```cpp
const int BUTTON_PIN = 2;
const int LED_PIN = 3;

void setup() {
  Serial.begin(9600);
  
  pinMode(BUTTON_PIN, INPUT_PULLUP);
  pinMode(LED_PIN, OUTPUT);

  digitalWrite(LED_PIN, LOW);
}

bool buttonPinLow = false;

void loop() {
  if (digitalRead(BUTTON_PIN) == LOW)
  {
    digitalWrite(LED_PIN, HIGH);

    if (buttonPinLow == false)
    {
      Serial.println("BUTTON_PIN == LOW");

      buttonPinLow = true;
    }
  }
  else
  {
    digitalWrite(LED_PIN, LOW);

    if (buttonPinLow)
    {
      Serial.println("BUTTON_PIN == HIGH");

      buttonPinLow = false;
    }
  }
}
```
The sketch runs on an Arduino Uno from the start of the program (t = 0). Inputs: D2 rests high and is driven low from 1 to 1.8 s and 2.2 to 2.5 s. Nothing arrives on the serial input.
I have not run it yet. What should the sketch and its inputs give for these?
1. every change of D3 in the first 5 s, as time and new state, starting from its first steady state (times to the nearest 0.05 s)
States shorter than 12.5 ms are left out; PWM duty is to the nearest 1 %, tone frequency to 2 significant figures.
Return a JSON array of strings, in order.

["0 s low; 1 s high; 1.8 s low; 2.2 s high; 2.5 s low"]
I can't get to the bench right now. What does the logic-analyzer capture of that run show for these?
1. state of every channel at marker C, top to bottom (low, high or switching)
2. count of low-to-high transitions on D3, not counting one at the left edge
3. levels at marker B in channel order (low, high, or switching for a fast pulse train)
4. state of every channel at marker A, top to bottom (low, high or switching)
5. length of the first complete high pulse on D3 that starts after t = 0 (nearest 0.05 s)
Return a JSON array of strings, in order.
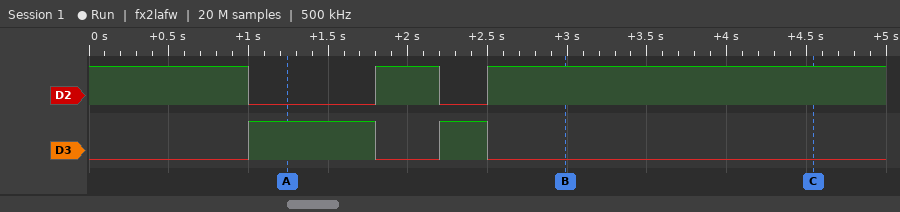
["D2 high, D3 low", "2", "D2 high, D3 low", "D2 low, D3 high", "0.80 s"]
